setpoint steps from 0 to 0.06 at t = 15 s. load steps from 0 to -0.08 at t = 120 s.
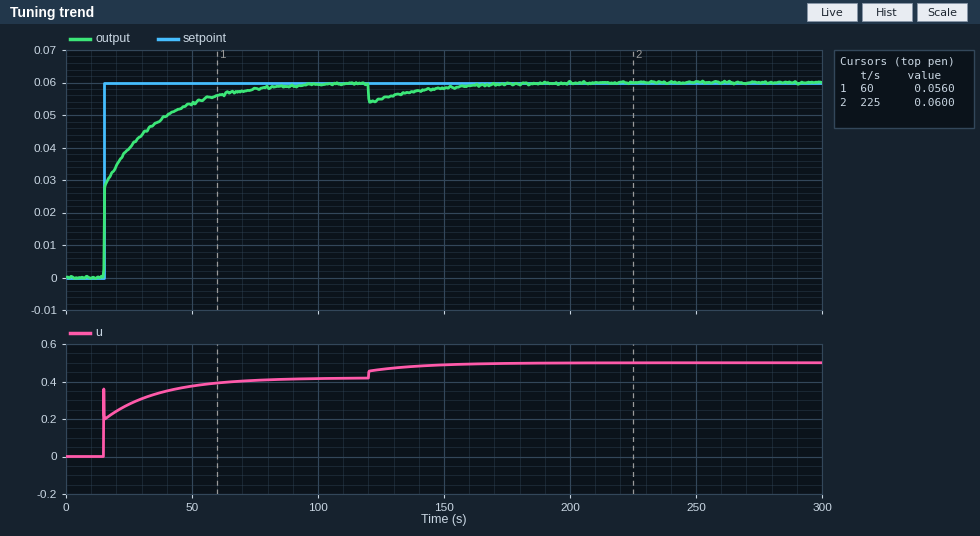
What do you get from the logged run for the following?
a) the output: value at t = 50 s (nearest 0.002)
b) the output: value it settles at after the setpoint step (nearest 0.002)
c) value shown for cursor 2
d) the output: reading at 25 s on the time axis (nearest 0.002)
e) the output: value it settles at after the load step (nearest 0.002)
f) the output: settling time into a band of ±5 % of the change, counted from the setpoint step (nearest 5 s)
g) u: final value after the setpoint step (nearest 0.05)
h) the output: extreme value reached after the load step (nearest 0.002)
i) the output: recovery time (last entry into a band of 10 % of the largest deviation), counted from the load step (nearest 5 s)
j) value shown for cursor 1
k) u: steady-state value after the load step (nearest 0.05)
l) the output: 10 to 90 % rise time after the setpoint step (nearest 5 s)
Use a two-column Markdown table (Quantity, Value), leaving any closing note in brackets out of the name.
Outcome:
| Quantity | Value |
|---|---|
| the output: value at t = 50 s | 0.054 |
| the output: value it settles at after the setpoint step | 0.060 |
| value shown for cursor 2 | 0.0600 |
| the output: reading at 25 s on the time axis | 0.040 |
| the output: value it settles at after the load step | 0.060 |
| the output: settling time into a band of ±5 % of the change, counted from the setpoint step | 50 s |
| u: final value after the setpoint step | 0.40 |
| the output: extreme value reached after the load step | 0.054 |
| the output: recovery time (last entry into a band of 10 % of the largest deviation), counted from the load step | 50 s |
| value shown for cursor 1 | 0.0560 |
| u: steady-state value after the load step | 0.50 |
| the output: 10 to 90 % rise time after the setpoint step | 35 s |
